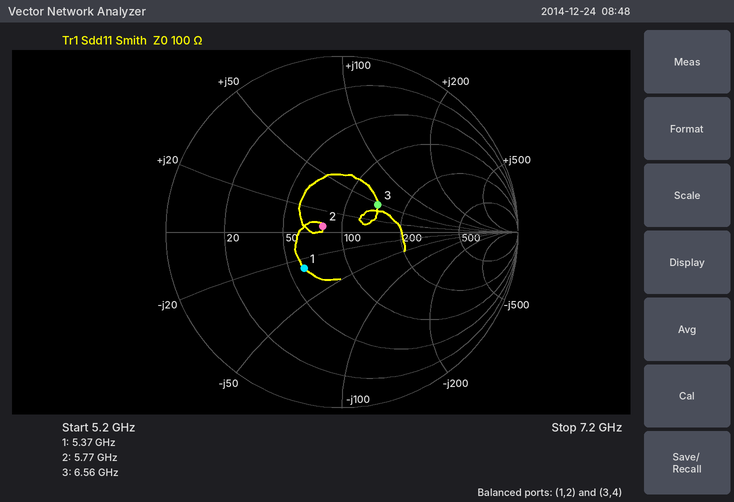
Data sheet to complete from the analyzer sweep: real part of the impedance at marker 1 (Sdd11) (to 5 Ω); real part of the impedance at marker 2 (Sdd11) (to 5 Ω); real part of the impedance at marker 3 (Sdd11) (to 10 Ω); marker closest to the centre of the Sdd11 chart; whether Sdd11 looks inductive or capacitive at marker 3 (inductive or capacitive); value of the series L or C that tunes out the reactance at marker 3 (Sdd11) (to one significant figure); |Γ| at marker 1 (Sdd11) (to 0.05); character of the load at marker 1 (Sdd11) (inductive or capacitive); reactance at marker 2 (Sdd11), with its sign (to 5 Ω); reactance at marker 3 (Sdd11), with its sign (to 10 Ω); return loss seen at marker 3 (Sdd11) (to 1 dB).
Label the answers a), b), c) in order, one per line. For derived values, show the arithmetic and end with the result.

a) 60 Ω
b) 80 Ω
c) 140 Ω
d) marker 2
e) inductive
f) C = 1/(2π × 6.56 GHz × 50 Ω) ≈ 485 fF, so 500 fF to one significant figure
g) 0.30
h) capacitive
i) +5 Ω
j) +50 Ω
k) 12 dB
